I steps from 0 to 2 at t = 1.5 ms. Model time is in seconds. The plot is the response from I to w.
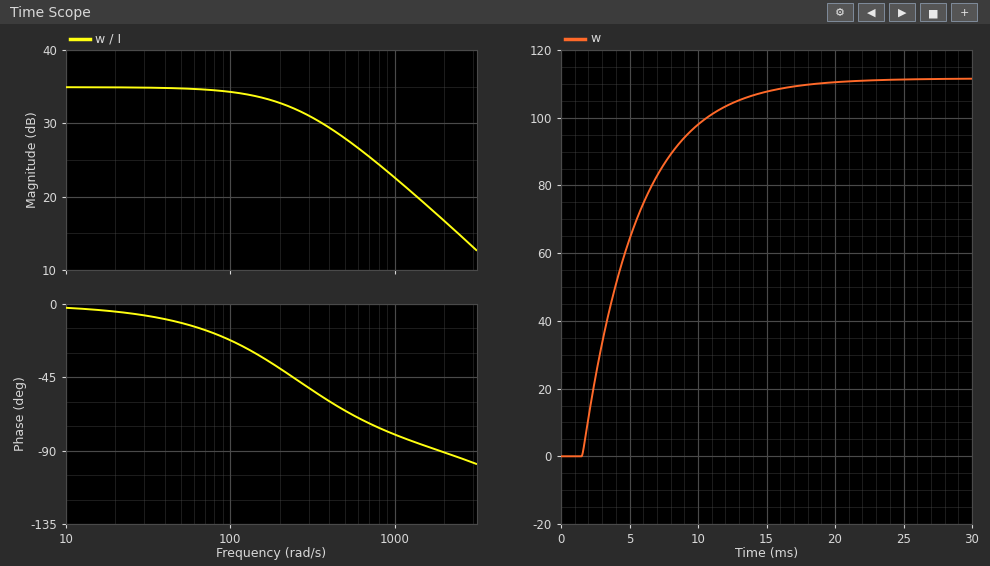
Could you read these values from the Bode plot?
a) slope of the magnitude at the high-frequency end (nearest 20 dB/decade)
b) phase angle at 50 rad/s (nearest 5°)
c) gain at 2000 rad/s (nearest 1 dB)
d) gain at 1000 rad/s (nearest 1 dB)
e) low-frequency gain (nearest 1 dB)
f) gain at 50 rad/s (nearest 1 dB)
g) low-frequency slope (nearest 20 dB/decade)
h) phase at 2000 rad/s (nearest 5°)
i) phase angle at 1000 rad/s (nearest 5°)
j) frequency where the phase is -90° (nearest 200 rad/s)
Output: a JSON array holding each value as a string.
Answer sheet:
["-20 dB/decade", "-10°", "17 dB", "23 dB", "35 dB", "35 dB", "0 dB/decade", "-90°", "-80°", "1800 rad/s"]
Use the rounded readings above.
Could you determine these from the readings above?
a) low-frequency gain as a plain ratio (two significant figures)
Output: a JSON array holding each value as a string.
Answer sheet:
["56"]
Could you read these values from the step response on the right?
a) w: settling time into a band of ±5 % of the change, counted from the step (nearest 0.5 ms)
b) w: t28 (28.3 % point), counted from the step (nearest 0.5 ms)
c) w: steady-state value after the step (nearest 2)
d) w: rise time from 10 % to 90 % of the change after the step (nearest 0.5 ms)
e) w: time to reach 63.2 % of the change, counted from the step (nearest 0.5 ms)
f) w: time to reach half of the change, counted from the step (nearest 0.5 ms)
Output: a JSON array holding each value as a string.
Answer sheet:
["12.0 ms", "1.5 ms", "112", "9.0 ms", "4.0 ms", "3.0 ms"]
